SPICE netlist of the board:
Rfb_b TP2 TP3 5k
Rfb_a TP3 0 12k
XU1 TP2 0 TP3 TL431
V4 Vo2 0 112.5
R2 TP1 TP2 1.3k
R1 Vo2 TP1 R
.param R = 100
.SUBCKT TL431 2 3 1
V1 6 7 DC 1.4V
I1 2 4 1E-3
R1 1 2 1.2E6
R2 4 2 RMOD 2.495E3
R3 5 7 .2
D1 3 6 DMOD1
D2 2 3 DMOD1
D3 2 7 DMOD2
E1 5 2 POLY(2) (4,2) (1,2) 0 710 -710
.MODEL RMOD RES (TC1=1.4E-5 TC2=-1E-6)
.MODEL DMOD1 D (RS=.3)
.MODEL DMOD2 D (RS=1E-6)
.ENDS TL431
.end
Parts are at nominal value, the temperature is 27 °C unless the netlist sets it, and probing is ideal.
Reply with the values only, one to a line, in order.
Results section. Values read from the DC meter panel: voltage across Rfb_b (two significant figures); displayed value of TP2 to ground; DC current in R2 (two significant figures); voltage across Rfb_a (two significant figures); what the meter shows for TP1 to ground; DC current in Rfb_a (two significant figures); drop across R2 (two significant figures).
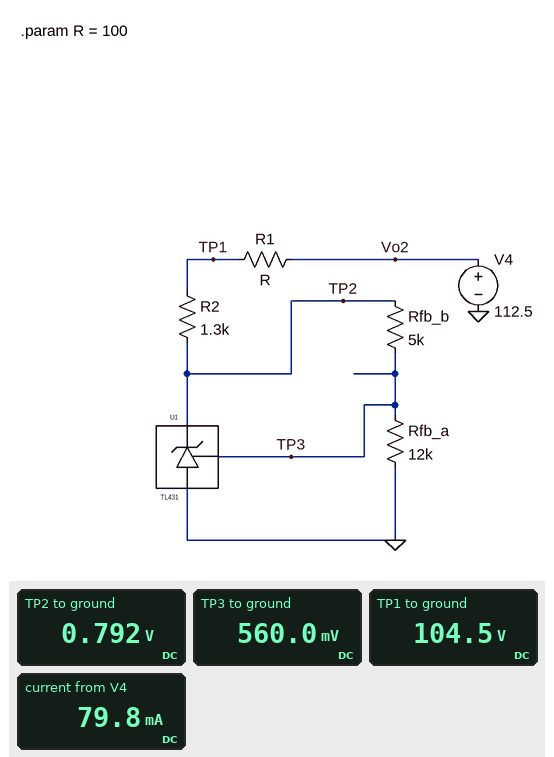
230 mV
0.792 V
80 mA
560 mV
104.5 V
47 µA
100 V
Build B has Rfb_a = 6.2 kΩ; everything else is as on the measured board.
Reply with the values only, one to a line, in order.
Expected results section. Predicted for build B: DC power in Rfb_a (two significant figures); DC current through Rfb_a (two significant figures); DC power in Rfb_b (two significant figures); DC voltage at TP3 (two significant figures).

31 µW
71 µA
25 µW
440 mV
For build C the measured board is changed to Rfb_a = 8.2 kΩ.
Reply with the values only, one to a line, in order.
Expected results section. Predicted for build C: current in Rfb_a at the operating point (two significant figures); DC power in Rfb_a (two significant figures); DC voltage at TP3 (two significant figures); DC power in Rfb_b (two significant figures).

60 µA
30 µW
490 mV
18 µW
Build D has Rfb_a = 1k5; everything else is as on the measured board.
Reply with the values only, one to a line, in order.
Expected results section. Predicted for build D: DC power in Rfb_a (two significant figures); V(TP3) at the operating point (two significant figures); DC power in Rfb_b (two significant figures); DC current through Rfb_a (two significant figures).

22 µW
180 mV
74 µW
120 µA
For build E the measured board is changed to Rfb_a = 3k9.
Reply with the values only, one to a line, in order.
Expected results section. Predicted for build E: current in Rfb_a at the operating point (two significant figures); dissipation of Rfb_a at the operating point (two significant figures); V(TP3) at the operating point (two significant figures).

89 µA
31 µW
350 mV
